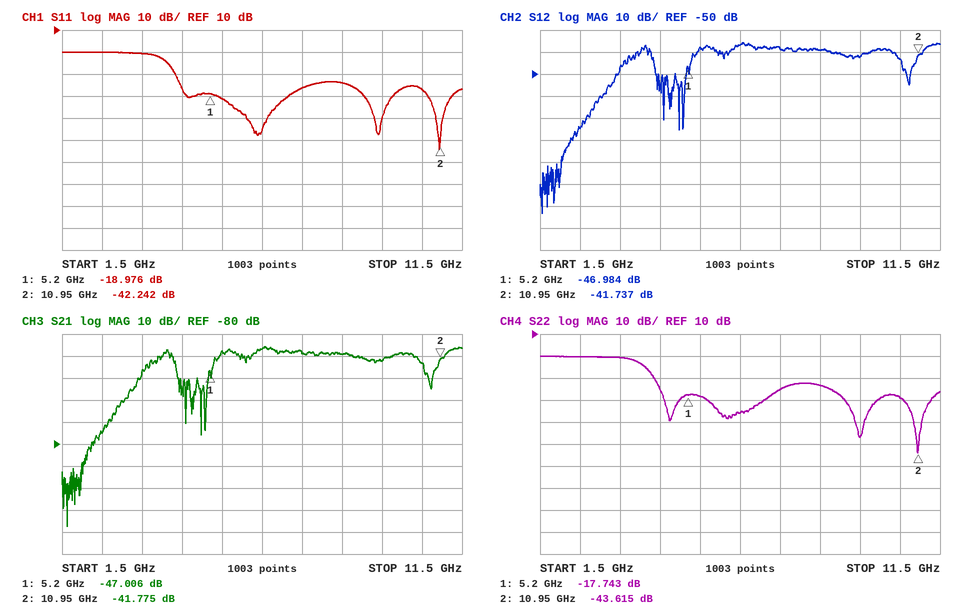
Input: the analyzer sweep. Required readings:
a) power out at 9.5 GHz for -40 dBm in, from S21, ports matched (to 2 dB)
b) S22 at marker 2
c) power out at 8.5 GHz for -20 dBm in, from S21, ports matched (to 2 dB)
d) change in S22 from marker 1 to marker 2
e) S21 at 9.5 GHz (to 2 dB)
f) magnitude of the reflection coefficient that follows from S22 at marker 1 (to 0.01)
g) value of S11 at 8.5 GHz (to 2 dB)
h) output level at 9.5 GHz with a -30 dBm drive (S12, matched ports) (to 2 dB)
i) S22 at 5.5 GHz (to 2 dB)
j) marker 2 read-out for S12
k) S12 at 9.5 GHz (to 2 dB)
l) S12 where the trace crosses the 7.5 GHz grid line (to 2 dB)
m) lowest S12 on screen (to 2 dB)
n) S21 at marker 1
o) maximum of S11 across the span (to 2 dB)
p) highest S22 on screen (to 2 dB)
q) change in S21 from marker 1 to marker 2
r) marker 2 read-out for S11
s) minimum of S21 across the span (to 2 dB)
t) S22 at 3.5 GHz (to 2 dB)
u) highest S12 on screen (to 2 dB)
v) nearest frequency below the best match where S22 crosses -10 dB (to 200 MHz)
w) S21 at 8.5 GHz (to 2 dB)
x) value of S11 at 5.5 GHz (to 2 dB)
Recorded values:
-82 dBm
-43.615 dB
-60 dBm
-25.872 dB
-42 dB
0.13
-14 dB
-72 dBm
-18 dB
-41.737 dB
-42 dB
-38 dB
-114 dB
-47.006 dB
0 dB
0 dB
5.231 dB
-42.242 dB
-118 dB
0 dB
-36 dB
4.4 GHz
-40 dB
-22 dB
